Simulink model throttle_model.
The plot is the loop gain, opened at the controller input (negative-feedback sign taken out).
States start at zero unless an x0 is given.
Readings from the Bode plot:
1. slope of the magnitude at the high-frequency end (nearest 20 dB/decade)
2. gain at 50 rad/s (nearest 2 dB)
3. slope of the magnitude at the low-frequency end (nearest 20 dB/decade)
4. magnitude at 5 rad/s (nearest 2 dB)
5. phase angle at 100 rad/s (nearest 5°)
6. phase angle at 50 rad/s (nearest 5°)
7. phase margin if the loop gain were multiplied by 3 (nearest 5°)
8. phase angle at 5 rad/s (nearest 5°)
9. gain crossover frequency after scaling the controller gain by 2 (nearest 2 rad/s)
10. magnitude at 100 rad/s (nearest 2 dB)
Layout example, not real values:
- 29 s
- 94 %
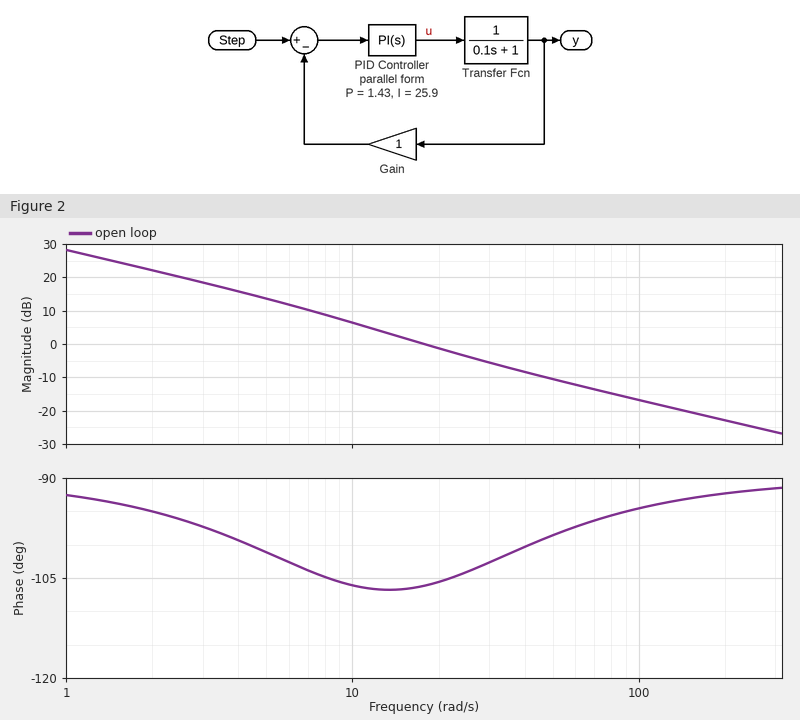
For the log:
- -20 dB/decade
- -10 dB
- -20 dB/decade
- 14 dB
- -95°
- -100°
- 80°
- -100°
- 32 rad/s
- -16 dB
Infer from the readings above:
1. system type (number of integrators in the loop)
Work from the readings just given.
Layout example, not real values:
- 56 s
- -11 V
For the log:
- 1
